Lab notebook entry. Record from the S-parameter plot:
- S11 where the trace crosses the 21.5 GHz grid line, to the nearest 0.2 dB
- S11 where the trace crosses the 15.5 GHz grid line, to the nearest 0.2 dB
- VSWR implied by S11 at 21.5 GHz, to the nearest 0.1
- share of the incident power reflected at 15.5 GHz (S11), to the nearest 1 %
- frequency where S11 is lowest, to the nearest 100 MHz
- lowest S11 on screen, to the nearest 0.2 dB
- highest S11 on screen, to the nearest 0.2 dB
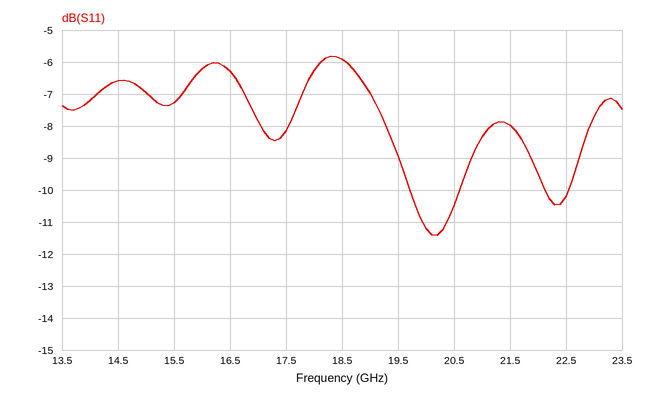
-8.0 dB
-7.2 dB
2.3
19 %
20.2 GHz
-11.4 dB
-5.8 dB
